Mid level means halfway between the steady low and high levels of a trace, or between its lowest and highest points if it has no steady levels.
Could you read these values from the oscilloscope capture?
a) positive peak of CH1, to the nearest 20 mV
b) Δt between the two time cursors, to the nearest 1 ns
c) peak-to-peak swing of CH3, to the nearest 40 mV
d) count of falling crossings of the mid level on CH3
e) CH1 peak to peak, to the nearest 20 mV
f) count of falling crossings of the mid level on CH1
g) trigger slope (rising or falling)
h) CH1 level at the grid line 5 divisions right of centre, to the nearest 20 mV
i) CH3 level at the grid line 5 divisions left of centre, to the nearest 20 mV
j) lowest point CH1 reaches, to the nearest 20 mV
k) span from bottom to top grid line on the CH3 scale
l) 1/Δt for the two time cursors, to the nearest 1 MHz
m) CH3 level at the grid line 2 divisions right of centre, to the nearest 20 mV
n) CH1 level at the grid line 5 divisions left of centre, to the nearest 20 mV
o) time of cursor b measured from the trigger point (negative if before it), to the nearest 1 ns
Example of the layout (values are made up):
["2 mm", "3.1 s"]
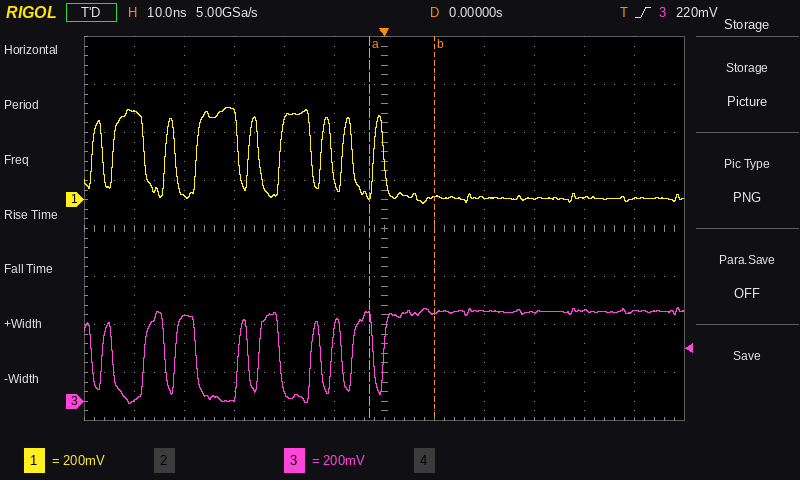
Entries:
["380 mV", "13 ns", "400 mV", "9", "400 mV", "9", "rising", "0 mV", "0 mV", "-20 mV", "1.6 V", "77 MHz", "380 mV", "360 mV", "+10 ns"]
